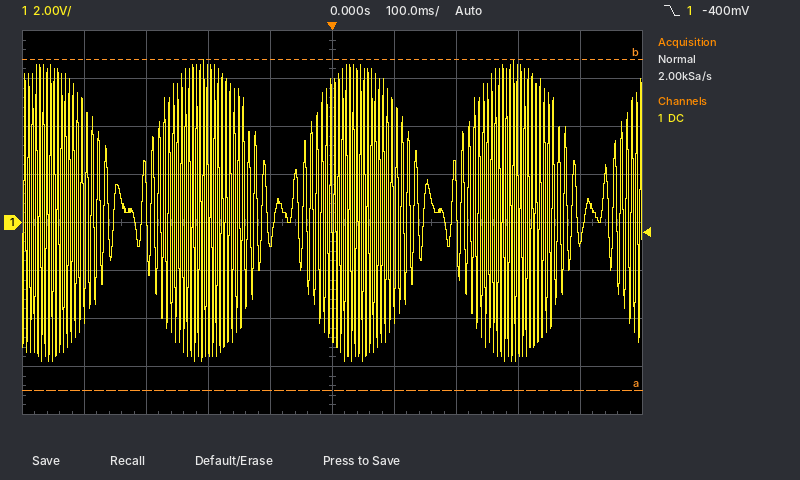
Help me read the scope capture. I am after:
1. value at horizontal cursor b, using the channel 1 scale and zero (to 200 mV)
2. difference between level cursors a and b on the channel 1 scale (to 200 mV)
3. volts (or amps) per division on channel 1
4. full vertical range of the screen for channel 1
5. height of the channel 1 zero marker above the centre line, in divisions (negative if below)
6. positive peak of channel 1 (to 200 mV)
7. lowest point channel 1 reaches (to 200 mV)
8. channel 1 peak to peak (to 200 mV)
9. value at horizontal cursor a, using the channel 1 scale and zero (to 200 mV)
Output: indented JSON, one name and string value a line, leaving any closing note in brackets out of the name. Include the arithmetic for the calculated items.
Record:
{
  "value at horizontal cursor b, using the channel 1 scale and zero": "6.8 V",
  "difference between level cursors a and b on the channel 1 scale": "13.8 V",
  "volts (or amps) per division on channel 1": "2 V",
  "full vertical range of the screen for channel 1": "16 V",
  "height of the channel 1 zero marker above the centre line, in divisions": "0.0 div",
  "positive peak of channel 1": "6.8 V",
  "lowest point channel 1 reaches": "-5.8 V",
  "channel 1 peak to peak": "6.8 V − (-5.8 V) = 12.6 V",
  "value at horizontal cursor a, using the channel 1 scale and zero": "-7.0 V"
}
